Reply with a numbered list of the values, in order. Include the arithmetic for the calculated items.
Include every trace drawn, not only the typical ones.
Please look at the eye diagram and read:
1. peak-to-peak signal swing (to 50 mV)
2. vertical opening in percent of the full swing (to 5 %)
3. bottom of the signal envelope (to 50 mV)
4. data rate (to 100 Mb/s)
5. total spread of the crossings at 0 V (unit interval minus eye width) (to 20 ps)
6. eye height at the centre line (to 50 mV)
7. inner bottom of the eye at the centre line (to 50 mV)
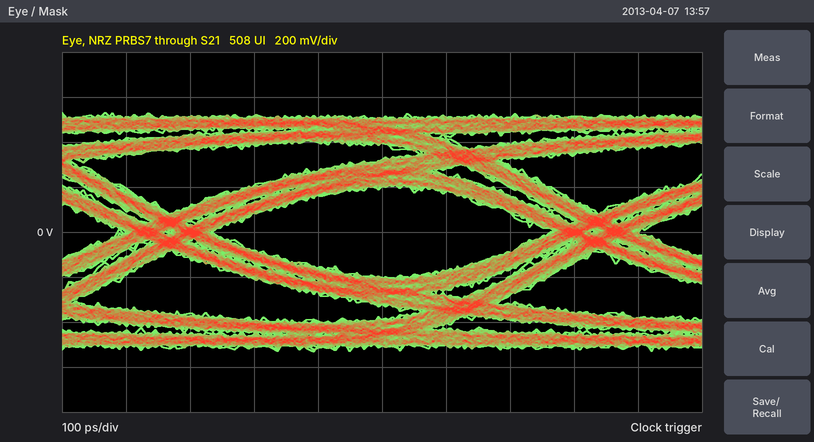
1. 1.05 V
2. 400 mV / 1.05 V ≈ 38.1 %, so 40 % to the nearest 5 %
3. -550 mV
4. 1.5 Gb/s
5. 140 ps
6. 400 mV
7. -200 mV
